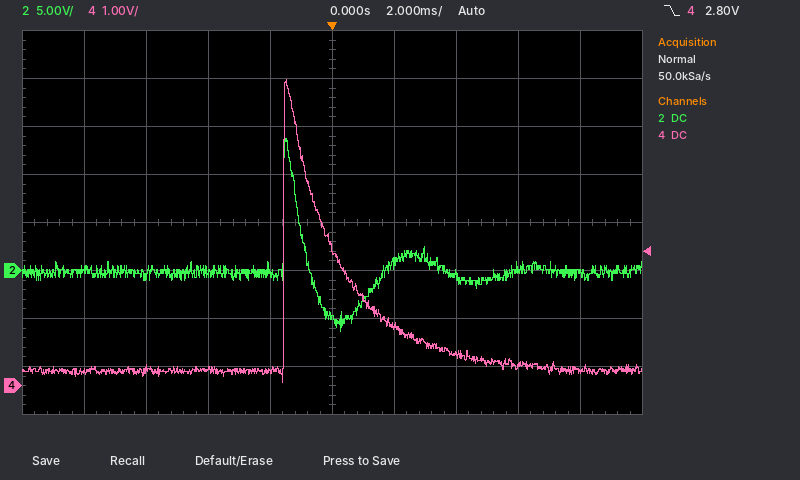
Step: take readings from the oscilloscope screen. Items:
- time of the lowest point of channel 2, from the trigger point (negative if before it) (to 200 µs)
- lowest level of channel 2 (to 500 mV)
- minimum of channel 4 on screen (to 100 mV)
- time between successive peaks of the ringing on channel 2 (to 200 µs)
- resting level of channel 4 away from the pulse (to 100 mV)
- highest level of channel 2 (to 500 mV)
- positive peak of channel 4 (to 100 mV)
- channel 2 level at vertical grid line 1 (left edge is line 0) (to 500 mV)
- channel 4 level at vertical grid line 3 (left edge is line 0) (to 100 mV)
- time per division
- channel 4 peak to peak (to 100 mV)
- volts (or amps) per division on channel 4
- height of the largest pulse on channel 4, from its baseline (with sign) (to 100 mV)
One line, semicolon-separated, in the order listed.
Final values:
+200 µs; -6.5 V; 100 mV; 4.0 ms; 300 mV; 14.0 V; 6.4 V; 0.0 V; 300 mV; 2 ms; 6.3 V; 1 V; +6.1 V
